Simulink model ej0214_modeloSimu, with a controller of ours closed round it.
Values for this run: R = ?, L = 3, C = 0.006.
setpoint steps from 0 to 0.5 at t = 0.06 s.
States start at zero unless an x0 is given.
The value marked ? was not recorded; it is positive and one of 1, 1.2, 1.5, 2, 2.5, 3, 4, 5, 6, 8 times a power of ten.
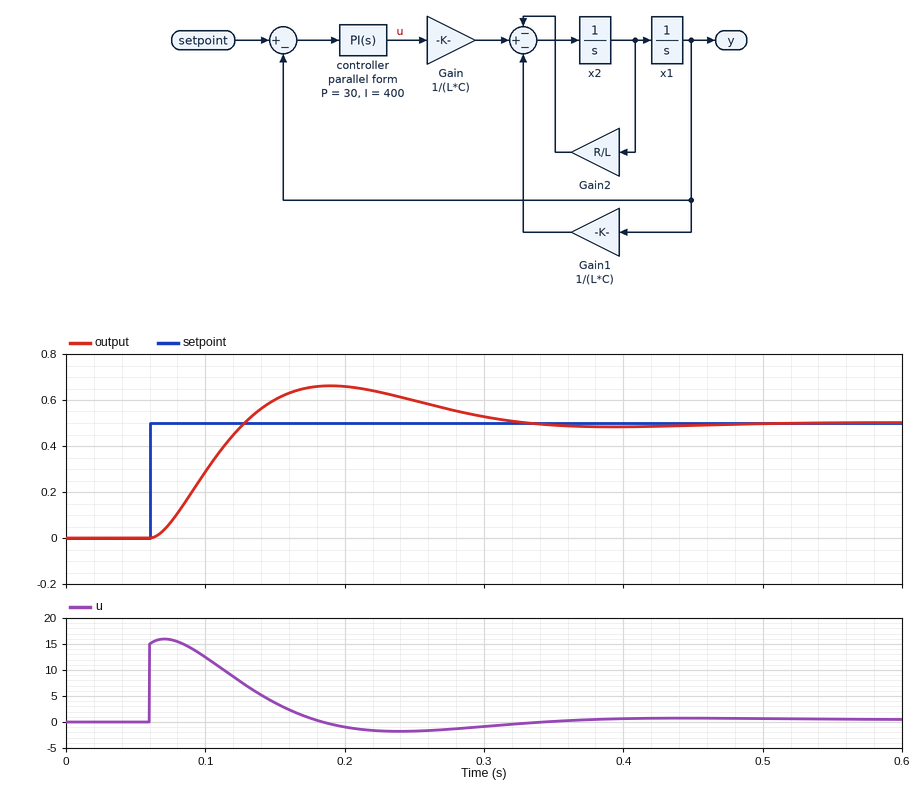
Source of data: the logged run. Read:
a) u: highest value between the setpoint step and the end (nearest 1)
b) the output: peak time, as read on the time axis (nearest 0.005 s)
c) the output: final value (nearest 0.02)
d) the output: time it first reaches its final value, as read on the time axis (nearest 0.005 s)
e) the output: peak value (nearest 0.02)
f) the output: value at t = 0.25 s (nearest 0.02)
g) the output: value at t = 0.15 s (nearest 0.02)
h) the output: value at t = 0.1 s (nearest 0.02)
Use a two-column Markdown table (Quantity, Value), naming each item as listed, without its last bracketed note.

| Quantity | Value |
|---|---|
| u: highest value between the setpoint step and the end | 16 |
| the output: peak time, as read on the time axis | 0.190 s |
| the output: final value | 0.50 |
| the output: time it first reaches its final value, as read on the time axis | 0.130 s |
| the output: peak value | 0.66 |
| the output: value at t = 0.25 s | 0.60 |
| the output: value at t = 0.15 s | 0.60 |
| the output: value at t = 0.1 s | 0.28 |
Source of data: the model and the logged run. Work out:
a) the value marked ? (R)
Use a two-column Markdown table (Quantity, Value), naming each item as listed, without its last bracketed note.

| Quantity | Value |
|---|---|
| the value marked ? | 250 |
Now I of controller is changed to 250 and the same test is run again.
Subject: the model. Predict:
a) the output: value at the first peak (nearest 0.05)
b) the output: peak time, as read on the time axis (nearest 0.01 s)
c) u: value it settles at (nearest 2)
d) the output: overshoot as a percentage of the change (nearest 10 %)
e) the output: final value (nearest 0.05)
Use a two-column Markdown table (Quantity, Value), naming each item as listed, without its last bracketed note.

| Quantity | Value |
|---|---|
| the output: value at the first peak | 0.60 |
| the output: peak time, as read on the time axis | 0.21 s |
| u: value it settles at | 0 |
| the output: overshoot as a percentage of the change | 20 % |
| the output: final value | 0.50 |
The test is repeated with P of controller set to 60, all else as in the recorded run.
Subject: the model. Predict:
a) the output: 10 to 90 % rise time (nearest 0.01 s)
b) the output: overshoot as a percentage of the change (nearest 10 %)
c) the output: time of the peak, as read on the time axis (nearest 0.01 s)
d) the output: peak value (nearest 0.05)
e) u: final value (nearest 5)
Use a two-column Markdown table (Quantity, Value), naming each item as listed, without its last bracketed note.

| Quantity | Value |
|---|---|
| the output: 10 to 90 % rise time | 0.03 s |
| the output: overshoot as a percentage of the change | 20 % |
| the output: time of the peak, as read on the time axis | 0.14 s |
| the output: peak value | 0.60 |
| u: final value | 0 |
